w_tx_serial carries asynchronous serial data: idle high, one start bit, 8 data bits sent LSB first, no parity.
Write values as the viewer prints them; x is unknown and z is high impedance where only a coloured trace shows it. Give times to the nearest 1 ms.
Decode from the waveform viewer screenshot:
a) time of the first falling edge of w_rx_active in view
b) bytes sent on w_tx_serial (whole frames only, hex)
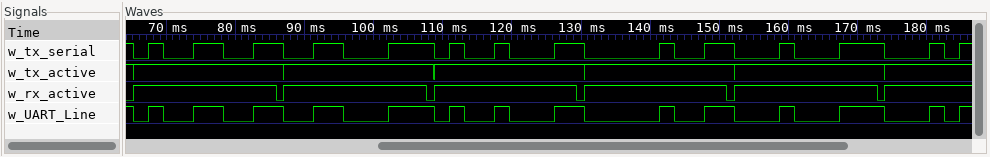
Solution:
86 ms
99, C6, 89, 90, C4
